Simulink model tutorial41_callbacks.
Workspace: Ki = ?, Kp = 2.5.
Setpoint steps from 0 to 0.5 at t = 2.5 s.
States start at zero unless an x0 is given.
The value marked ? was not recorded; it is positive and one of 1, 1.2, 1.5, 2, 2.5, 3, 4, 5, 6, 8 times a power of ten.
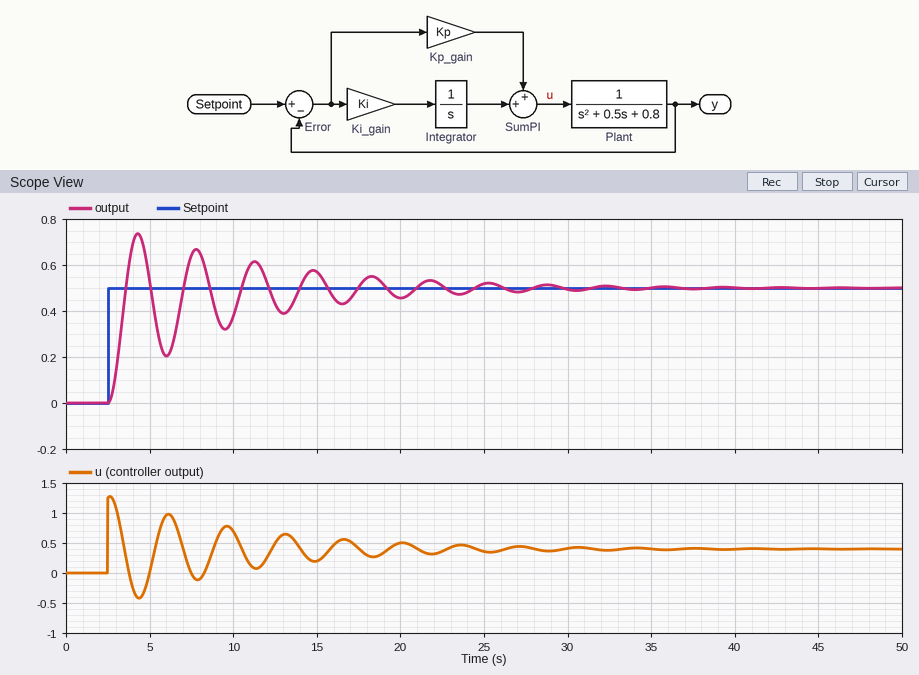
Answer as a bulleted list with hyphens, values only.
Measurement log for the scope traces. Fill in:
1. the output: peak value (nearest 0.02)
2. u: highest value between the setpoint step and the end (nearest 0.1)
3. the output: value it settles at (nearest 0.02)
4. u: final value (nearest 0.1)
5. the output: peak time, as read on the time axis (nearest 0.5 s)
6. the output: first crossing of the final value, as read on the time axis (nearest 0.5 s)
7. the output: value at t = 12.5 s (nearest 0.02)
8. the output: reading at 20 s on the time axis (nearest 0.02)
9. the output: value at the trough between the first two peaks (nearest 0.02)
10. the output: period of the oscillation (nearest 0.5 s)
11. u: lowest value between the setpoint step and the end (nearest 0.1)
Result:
- 0.74
- 1.3
- 0.50
- 0.4
- 4.5 s
- 3.5 s
- 0.44
- 0.46
- 0.20
- 3.5 s
- -0.4
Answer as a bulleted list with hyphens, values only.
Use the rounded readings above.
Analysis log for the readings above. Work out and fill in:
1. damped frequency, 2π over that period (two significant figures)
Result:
- 1.8 rad/s
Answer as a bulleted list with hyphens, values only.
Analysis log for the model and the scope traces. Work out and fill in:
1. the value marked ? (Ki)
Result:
- 0.8
